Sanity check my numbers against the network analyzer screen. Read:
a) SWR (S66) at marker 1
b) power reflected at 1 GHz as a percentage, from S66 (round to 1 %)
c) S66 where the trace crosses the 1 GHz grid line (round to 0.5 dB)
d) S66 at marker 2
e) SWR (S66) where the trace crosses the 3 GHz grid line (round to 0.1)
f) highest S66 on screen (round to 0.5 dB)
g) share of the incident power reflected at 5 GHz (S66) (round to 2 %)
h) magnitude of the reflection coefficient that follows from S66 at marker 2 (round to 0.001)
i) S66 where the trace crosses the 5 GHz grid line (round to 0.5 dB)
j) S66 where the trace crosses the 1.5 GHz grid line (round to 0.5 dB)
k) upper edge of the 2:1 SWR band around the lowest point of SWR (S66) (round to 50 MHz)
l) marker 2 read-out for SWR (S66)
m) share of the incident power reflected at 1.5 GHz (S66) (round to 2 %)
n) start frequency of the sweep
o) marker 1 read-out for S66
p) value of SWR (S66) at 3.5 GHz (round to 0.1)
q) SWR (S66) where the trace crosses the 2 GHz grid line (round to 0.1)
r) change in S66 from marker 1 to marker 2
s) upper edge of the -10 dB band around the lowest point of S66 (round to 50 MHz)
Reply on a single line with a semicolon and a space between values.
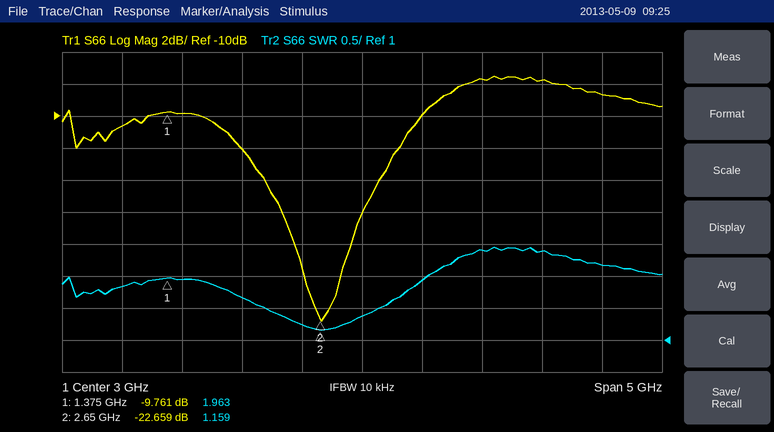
1.963; 9 %; -10.5 dB; -22.659 dB; 1.4; -7.5 dB; 14 %; 0.074; -8.5 dB; -10.0 dB; 3.55 GHz; 1.159; 10 %; 500 MHz; -9.761 dB; 1.9; 1.7; -12.898 dB; 3.50 GHz
